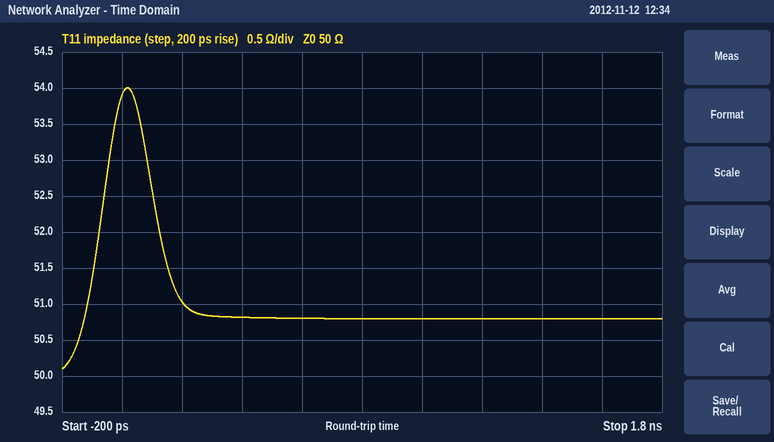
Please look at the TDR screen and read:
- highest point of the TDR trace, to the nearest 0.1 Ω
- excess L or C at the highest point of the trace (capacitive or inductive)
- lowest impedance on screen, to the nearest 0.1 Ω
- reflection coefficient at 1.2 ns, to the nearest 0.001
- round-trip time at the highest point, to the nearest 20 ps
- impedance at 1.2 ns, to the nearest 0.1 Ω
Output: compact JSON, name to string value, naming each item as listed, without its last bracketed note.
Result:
{"highest point of the TDR trace, to the nearest 0.1 Ω": "54.0 Ω", "excess L or C at the highest point of the trace": "inductive", "lowest impedance on screen, to the nearest 0.1 Ω": "50.1 Ω", "reflection coefficient at 1.2 ns, to the nearest 0.001": "+0.008", "round-trip time at the highest point, to the nearest 20 ps": "20 ps", "impedance at 1.2 ns, to the nearest 0.1 Ω": "50.8 Ω"}
